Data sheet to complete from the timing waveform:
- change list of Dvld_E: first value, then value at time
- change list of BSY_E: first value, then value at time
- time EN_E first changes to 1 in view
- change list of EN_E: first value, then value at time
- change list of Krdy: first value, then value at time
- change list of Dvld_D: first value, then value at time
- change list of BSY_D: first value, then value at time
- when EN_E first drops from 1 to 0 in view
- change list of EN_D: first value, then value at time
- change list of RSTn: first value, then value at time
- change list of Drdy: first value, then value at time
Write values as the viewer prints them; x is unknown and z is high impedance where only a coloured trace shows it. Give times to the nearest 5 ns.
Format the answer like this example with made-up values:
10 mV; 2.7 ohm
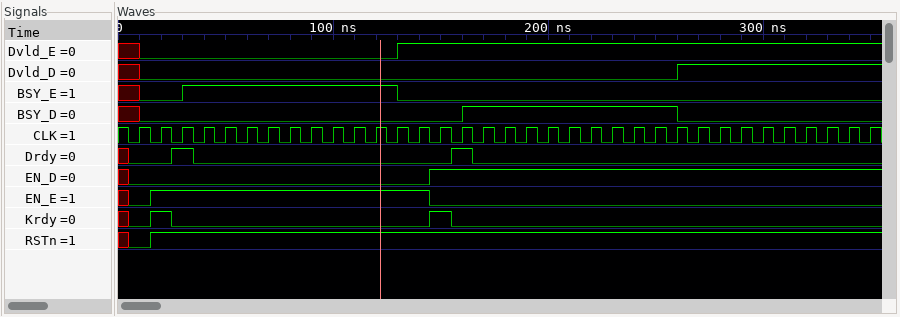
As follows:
x, 0 at 10 ns, 1 at 130 ns; x, 0 at 10 ns, 1 at 30 ns, 0 at 130 ns; 15 ns; x, 0 at 5 ns, 1 at 15 ns, 0 at 145 ns; x, 0 at 5 ns, 1 at 15 ns, 0 at 25 ns, 1 at 145 ns, 0 at 155 ns; x, 0 at 10 ns, 1 at 260 ns; x, 0 at 10 ns, 1 at 160 ns, 0 at 260 ns; 145 ns; x, 0 at 5 ns, 1 at 145 ns; x, 0 at 5 ns, 1 at 15 ns; x, 0 at 5 ns, 1 at 25 ns, 0 at 35 ns, 1 at 155 ns, 0 at 165 ns
